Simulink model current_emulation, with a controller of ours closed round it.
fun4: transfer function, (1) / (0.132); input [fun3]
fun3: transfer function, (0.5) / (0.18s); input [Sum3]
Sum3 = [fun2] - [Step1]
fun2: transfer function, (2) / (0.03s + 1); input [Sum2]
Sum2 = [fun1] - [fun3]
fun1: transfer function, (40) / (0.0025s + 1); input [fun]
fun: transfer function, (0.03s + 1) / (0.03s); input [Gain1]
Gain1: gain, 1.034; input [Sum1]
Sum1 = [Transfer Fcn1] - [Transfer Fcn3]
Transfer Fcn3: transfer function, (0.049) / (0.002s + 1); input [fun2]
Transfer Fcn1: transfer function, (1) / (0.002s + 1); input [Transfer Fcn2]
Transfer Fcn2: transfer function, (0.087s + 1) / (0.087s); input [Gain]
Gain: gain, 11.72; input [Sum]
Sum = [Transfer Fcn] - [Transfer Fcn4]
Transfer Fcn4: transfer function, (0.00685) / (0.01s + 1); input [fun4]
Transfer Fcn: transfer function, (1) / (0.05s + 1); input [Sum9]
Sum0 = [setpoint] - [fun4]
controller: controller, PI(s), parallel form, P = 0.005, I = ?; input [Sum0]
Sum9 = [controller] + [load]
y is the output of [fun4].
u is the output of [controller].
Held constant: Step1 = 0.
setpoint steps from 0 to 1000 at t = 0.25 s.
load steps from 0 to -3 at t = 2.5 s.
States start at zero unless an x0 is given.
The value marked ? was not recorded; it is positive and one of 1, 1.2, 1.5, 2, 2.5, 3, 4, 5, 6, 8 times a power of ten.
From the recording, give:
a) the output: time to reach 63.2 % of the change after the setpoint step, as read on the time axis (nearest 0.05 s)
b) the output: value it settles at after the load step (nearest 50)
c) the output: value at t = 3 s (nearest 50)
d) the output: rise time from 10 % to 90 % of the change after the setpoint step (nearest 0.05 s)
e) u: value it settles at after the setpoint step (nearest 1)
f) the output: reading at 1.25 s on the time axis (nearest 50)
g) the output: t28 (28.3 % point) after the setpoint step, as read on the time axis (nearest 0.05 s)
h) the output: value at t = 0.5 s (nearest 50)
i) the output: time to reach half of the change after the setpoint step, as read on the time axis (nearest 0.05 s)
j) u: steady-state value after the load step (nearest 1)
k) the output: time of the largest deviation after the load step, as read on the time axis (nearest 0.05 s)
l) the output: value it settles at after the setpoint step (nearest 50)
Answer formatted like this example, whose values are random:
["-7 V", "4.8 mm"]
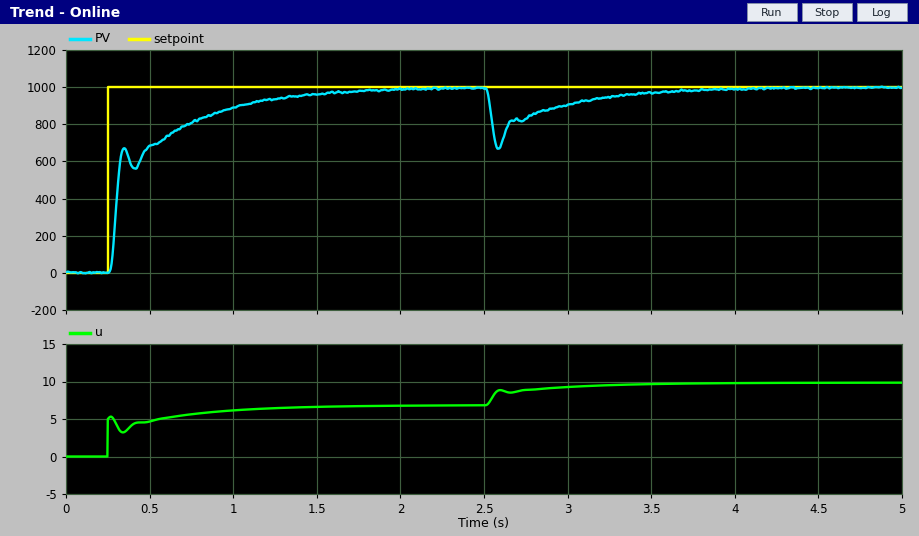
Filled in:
["0.35 s", "1000", "900", "0.75 s", "7", "950", "0.30 s", "700", "0.30 s", "10", "2.60 s", "1000"]
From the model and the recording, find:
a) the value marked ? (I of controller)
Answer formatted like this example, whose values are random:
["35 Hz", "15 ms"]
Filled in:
["0.025"]
